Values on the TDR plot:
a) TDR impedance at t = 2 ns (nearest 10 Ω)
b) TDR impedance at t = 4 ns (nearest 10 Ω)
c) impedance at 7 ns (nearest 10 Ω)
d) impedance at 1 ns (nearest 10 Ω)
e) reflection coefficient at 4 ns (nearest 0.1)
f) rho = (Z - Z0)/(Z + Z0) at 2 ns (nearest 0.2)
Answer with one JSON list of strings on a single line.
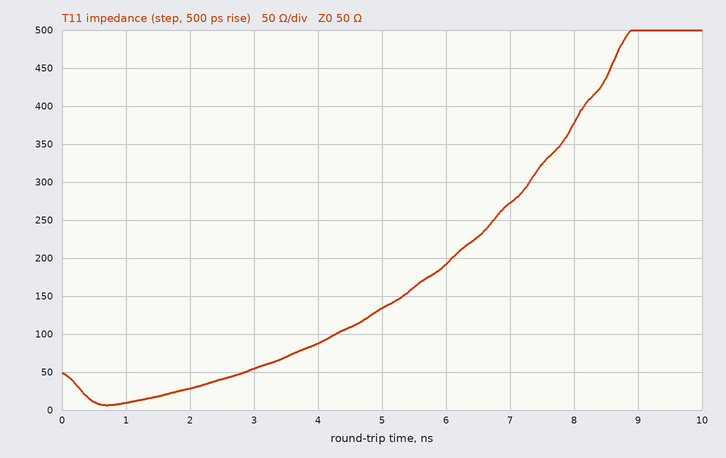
["30 Ω", "90 Ω", "270 Ω", "10 Ω", "+0.3", "-0.2"]
